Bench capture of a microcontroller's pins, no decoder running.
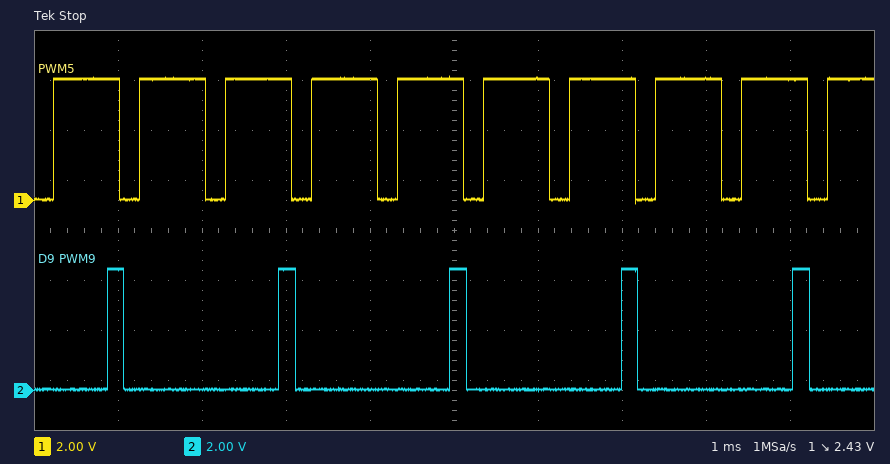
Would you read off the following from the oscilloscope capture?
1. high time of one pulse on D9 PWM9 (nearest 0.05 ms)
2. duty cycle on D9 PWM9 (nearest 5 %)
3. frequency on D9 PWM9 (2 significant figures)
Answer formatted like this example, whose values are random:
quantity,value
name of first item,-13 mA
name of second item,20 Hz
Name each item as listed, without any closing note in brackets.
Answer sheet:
quantity,value
high time of one pulse on D9 PWM9,0.20 ms
duty cycle on D9 PWM9,10 %
frequency on D9 PWM9,490 Hz
